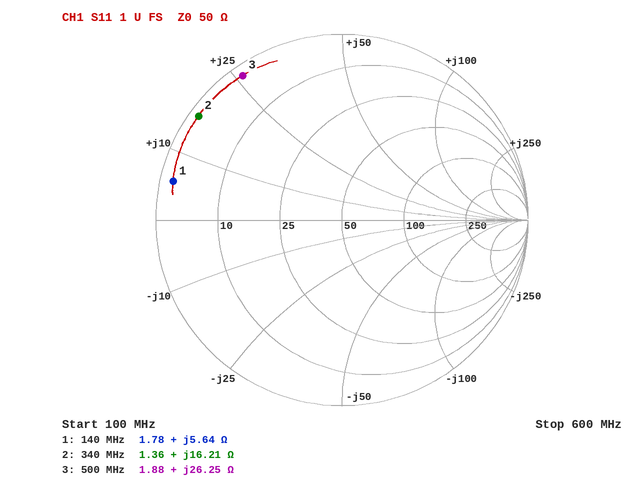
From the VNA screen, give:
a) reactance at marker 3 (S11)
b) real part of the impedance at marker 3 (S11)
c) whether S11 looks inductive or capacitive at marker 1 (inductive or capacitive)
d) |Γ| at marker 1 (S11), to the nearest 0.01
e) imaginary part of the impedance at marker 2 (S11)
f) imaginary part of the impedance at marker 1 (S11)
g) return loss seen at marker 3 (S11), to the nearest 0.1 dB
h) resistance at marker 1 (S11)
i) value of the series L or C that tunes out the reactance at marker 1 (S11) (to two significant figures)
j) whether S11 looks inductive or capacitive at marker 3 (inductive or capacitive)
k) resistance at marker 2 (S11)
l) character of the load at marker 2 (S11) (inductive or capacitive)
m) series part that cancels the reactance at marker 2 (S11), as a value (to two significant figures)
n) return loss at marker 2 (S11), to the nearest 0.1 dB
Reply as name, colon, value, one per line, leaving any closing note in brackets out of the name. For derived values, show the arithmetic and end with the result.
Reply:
reactance at marker 3: +26.25 Ω
real part of the impedance at marker 3: 1.88 Ω
whether S11 looks inductive or capacitive at marker 1: inductive
|Γ| at marker 1 (S11), to the nearest 0.01: 0.93
imaginary part of the impedance at marker 2: +16.21 Ω
imaginary part of the impedance at marker 1: +5.64 Ω
return loss seen at marker 3 (S11), to the nearest 0.1 dB: 0.5 dB
resistance at marker 1: 1.78 Ω
value of the series L or C that tunes out the reactance at marker 1 (S11): C = 1/(2π × 140 MHz × 5.64 Ω) ≈ 202 pF, so 200 pF to two significant figures
whether S11 looks inductive or capacitive at marker 3: inductive
resistance at marker 2: 1.36 Ω
character of the load at marker 2 (S11): inductive
series part that cancels the reactance at marker 2 (S11), as a value: C = 1/(2π × 340 MHz × 16.21 Ω) ≈ 29 pF
return loss at marker 2 (S11), to the nearest 0.1 dB: 0.4 dB
